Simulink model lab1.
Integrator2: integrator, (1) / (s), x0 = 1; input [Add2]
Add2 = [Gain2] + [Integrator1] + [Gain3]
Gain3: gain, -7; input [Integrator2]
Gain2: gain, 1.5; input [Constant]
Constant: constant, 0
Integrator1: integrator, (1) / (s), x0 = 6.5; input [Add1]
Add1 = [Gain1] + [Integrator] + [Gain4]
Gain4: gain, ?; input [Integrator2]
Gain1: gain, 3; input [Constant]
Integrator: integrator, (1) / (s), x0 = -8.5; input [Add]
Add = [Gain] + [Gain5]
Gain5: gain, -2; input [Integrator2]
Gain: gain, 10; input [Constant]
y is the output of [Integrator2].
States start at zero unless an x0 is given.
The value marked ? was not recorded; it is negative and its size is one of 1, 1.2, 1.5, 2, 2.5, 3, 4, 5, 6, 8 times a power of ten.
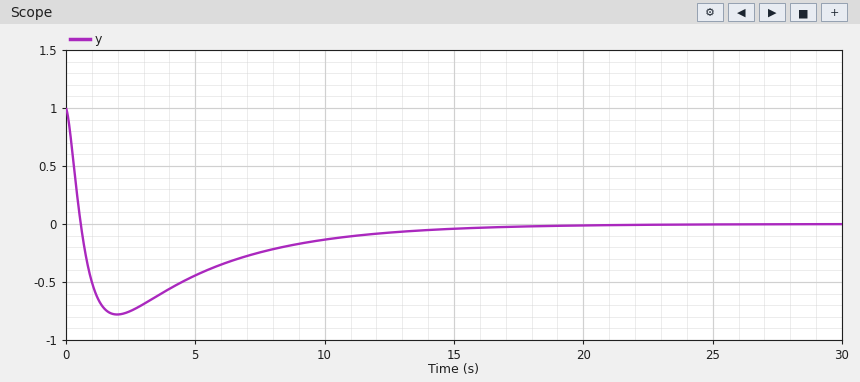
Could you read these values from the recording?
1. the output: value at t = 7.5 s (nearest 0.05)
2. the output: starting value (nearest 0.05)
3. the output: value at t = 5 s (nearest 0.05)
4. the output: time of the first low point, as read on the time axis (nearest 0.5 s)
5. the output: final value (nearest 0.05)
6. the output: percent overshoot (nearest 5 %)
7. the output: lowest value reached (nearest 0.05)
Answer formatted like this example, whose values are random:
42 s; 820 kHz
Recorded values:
-0.25; 1.00; -0.45; 2.0 s; 0.00; 80 %; -0.80
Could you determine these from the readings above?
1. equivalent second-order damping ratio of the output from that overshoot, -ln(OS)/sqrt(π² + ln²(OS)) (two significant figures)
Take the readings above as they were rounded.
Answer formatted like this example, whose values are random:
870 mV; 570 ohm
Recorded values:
0.071
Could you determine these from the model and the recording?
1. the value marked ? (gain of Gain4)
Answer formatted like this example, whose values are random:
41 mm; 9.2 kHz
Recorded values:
-10
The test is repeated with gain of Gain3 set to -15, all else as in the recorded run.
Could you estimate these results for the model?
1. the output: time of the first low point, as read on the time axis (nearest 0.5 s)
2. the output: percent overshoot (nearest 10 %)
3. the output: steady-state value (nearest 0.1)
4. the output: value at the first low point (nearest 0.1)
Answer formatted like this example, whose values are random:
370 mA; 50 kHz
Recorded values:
3.5 s; 60 %; 0.0; -0.6
